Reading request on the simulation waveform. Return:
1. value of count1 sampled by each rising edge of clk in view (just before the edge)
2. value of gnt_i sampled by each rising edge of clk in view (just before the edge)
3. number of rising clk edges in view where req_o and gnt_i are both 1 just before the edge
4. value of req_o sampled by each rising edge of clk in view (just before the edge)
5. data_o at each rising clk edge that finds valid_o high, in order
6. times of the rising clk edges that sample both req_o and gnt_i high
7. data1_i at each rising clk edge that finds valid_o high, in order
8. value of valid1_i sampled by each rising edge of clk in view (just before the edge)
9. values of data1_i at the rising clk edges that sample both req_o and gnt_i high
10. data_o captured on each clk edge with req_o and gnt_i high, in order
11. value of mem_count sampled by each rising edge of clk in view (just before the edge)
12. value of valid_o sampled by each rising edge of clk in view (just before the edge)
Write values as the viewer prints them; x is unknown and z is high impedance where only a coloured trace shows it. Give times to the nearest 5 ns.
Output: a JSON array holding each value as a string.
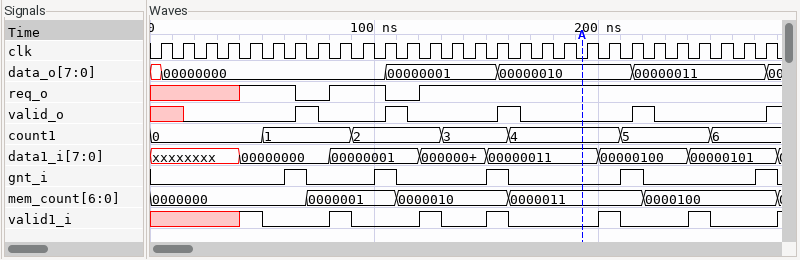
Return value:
["0, 0, 0, 0, 0, 1, 1, 1, 1, 2, 2, 2, 2, 3, 3, 3, 4, 4, 4, 4, 4, 5, 5, 5, 5, 6, 6, 6", "0 0 0 0 0 0 1 0 0 0 1 0 0 0 0 1 0 0 0 0 0 1 0 0 0 0 0 1", "5", "x x x x 1 1 1 0 1 1 1 0 1 1 1 1 1 1 1 1 1 1 1 1 1 1 1 1", "00000000, 00000001, 00000010, 00000011", "65 ns, 105 ns, 155 ns, 215 ns, 275 ns", "00000000, 00000001, 00000011, 00000100", "x x x x 1 0 0 0 1 0 0 0 1 0 0 1 0 0 0 0 1 0 0 0 1 0 0 0", "00000000, 00000001, 00000011, 00000100, 00000101", "00000000, 00000000, 00000001, 00000010, 00000011", "0000000, 0000000, 0000000, 0000000, 0000000, 0000000, 0000000, 0000001, 0000001, 0000001, 0000001, 0000010, 0000010, 0000010, 0000010, 0000010, 0000011, 0000011, 0000011, 0000011, 0000011, 0000011, 0000100, 0000100, 0000100, 0000100, 0000100, 0000100", "x x 0 0 0 0 0 1 0 0 0 1 0 0 0 0 1 0 0 0 0 0 1 0 0 0 0 0"]
